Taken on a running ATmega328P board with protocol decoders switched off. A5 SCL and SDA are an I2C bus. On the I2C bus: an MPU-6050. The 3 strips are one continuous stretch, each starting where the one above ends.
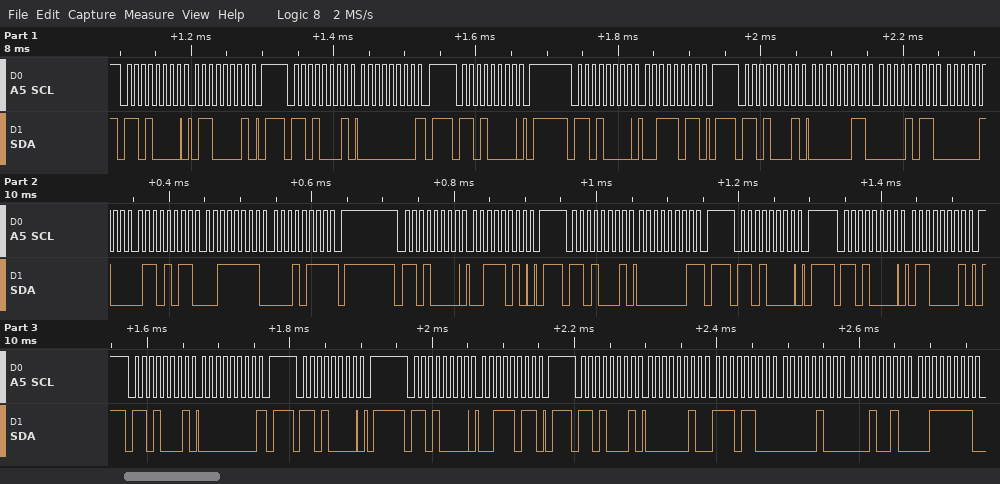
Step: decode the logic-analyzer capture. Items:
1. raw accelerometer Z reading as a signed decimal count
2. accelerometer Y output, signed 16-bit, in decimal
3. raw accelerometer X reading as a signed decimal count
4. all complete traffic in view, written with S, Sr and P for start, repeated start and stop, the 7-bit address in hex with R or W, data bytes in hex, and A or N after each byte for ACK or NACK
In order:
16151
1131
779
S 68W A 61 A P S 68R A 00 N P S 68W A P S 68W A 3B A P S 68R A 03 A 0B A 04 A 6B A 3F A 17 N P S 68W A 3A A P S 68R A 01 N P S 68W A P S 68W A 61 A P S 68R A 00 N P S 68W A P S 68W A 3B A P S 68R A 02 A EC A 04 A 12 A 3F A
